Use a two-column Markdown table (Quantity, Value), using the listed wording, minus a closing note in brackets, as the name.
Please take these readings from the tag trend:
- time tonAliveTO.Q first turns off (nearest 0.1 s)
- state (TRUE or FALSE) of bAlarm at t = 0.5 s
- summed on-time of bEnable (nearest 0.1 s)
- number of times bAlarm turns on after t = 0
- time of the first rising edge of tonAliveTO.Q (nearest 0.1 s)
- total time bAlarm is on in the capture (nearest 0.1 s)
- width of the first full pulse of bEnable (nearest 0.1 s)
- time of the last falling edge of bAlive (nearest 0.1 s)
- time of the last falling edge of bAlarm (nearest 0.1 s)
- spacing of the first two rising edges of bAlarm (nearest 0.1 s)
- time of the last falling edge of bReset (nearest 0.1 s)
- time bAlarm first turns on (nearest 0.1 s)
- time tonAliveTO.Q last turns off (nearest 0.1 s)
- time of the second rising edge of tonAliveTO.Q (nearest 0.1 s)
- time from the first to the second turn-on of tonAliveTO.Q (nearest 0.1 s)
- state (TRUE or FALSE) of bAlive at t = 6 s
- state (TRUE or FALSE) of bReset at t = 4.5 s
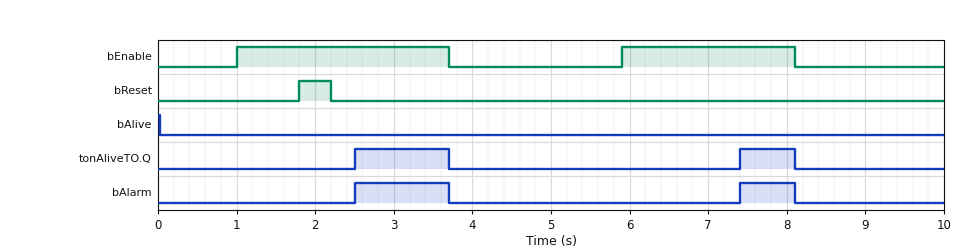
| Quantity | Value |
|---|---|
| time tonAliveTO.Q first turns off | 3.7 s |
| state (TRUE or FALSE) of bAlarm at t = 0.5 s | FALSE |
| summed on-time of bEnable | 4.9 s |
| number of times bAlarm turns on after t = 0 | 2 |
| time of the first rising edge of tonAliveTO.Q | 2.5 s |
| total time bAlarm is on in the capture | 1.9 s |
| width of the first full pulse of bEnable | 2.7 s |
| time of the last falling edge of bAlive | 0.0 s |
| time of the last falling edge of bAlarm | 8.1 s |
| spacing of the first two rising edges of bAlarm | 4.9 s |
| time of the last falling edge of bReset | 2.2 s |
| time bAlarm first turns on | 2.5 s |
| time tonAliveTO.Q last turns off | 8.1 s |
| time of the second rising edge of tonAliveTO.Q | 7.4 s |
| time from the first to the second turn-on of tonAliveTO.Q | 4.9 s |
| state (TRUE or FALSE) of bAlive at t = 6 s | FALSE |
| state (TRUE or FALSE) of bReset at t = 4.5 s | FALSE |
